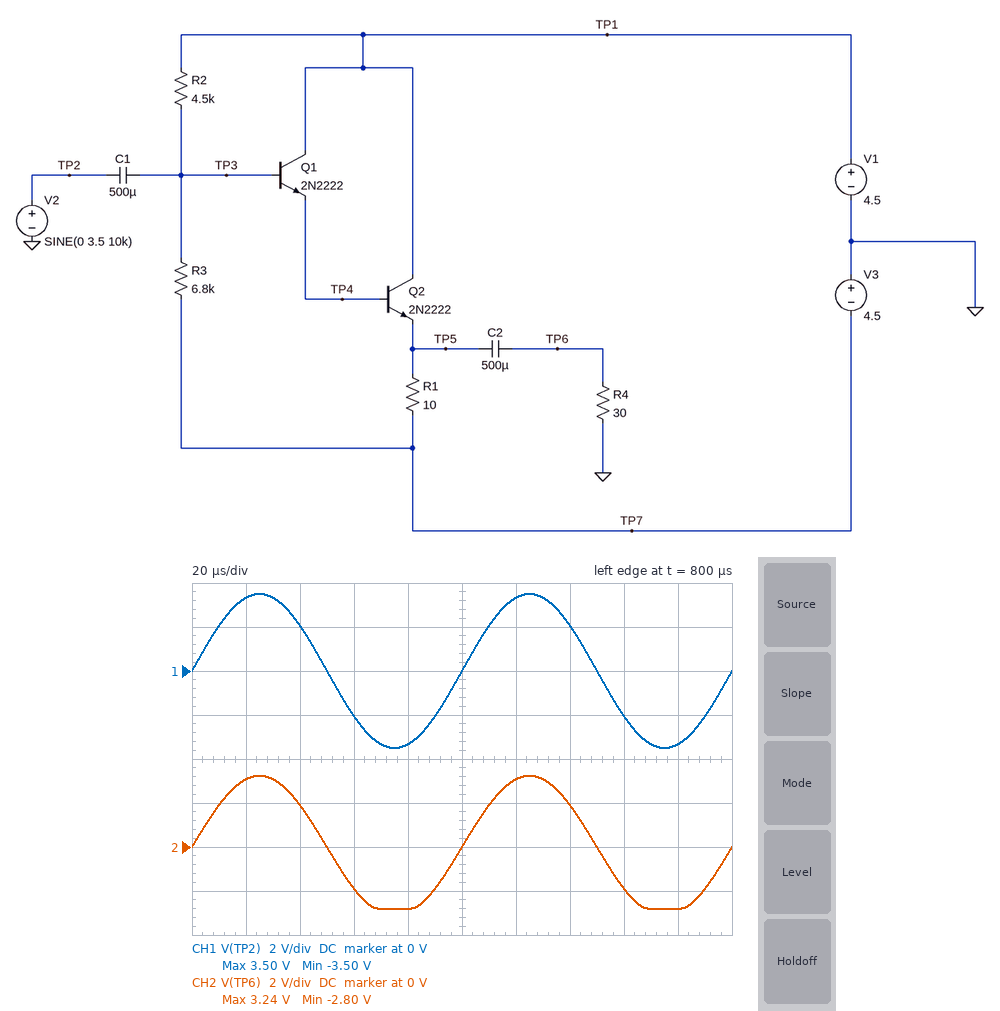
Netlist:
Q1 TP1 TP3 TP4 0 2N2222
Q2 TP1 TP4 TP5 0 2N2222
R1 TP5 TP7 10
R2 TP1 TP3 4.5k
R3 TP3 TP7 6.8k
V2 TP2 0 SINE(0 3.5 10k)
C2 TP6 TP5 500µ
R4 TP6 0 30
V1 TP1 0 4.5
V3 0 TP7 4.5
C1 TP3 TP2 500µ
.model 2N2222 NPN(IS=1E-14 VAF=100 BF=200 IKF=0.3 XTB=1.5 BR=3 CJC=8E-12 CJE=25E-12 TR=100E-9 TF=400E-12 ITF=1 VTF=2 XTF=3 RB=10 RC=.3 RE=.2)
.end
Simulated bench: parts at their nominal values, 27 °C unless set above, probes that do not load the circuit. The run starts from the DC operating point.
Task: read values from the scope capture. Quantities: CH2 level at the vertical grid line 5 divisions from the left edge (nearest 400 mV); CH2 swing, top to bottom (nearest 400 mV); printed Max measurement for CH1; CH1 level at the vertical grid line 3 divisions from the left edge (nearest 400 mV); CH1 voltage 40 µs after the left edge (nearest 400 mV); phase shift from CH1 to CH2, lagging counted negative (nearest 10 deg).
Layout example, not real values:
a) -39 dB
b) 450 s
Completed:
a) 0 V
b) 6.0 V
c) 3.50 V
d) -2.0 V
e) 2.0 V
f) 0 deg
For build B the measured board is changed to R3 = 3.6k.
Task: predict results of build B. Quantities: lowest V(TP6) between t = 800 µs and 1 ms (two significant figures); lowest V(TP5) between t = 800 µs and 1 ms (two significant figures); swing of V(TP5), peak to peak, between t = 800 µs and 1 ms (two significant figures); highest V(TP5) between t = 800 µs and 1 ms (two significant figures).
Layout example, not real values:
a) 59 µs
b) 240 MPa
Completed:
a) -1.8 V
b) -3.9 V
c) 5.1 V
d) 1.2 V
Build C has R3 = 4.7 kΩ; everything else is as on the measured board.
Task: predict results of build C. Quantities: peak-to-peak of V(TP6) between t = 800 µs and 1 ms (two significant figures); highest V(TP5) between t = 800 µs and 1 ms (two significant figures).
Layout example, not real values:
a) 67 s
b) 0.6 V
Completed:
a) 5.5 V
b) 1.7 V
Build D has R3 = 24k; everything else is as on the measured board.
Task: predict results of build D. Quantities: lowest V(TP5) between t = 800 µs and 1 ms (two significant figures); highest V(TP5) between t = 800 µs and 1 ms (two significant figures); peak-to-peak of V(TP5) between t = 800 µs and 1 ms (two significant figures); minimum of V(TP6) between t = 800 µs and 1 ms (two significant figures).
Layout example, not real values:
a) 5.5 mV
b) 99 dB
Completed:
a) -2.1 V
b) 3.3 V
c) 5.4 V
d) -3.3 V
